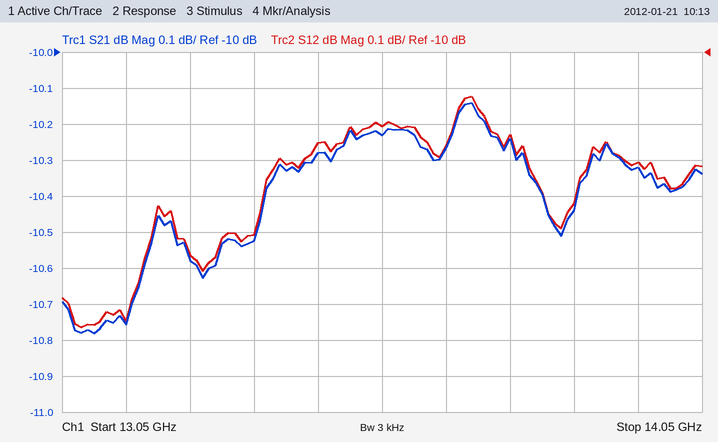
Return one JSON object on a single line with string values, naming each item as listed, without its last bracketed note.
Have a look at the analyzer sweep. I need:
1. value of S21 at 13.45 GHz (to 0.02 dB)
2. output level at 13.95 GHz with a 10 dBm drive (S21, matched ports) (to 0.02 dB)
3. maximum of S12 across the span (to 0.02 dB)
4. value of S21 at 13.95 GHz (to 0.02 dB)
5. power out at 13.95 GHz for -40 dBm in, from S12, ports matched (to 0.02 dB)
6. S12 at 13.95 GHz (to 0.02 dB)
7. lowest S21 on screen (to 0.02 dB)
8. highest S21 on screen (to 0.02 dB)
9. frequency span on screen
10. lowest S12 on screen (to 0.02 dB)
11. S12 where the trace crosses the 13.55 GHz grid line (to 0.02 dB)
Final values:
{"value of S21 at 13.45 GHz": "-10.28 dB", "output level at 13.95 GHz with a 10 dBm drive (S21, matched ports)": "-0.32 dBm", "maximum of S12 across the span": "-10.12 dB", "value of S21 at 13.95 GHz": "-10.32 dB", "power out at 13.95 GHz for -40 dBm in, from S12, ports matched": "-50.30 dBm", "S12 at 13.95 GHz": "-10.30 dB", "lowest S21 on screen": "-10.78 dB", "highest S21 on screen": "-10.14 dB", "frequency span on screen": "1 GHz", "lowest S12 on screen": "-10.76 dB", "S12 where the trace crosses the 13.55 GHz grid line": "-10.20 dB"}
